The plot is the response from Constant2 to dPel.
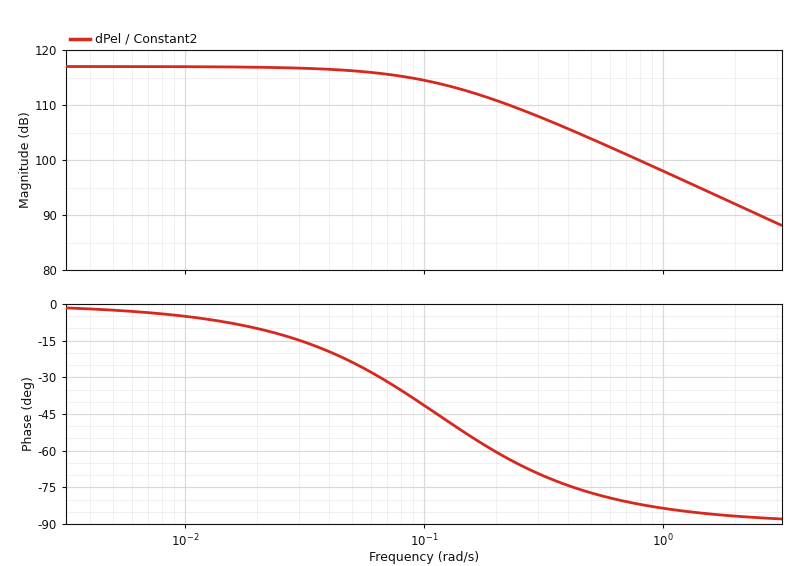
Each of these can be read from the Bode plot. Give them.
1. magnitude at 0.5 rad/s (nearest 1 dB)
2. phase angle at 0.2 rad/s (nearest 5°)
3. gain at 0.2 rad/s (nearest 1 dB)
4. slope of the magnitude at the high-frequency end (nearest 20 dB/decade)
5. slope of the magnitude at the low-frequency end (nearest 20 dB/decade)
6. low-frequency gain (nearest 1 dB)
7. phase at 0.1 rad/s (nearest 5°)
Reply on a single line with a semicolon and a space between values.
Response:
104 dB; -60°; 111 dB; -20 dB/decade; 0 dB/decade; 117 dB; -40°
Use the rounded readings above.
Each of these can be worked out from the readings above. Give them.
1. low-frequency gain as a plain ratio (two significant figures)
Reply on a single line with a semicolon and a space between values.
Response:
710000
